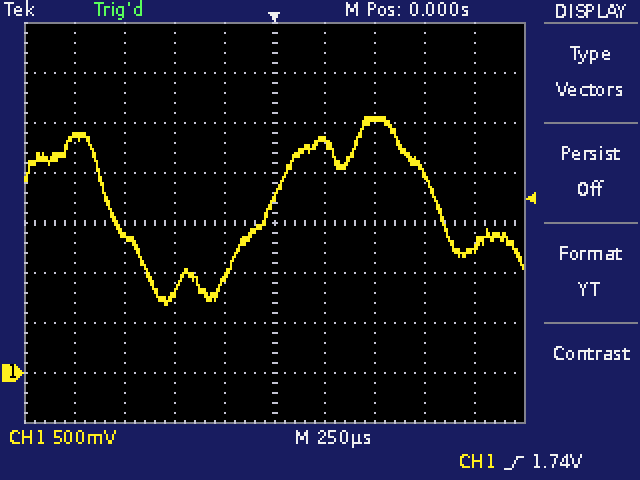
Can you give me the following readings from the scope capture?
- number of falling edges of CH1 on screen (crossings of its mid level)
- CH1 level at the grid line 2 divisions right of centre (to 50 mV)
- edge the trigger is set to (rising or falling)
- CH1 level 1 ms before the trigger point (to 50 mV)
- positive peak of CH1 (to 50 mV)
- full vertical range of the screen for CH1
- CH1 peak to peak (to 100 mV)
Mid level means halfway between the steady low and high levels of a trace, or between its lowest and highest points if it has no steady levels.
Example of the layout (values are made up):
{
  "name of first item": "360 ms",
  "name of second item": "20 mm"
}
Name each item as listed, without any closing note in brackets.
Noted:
{
  "number of falling edges of CH1 on screen": "2",
  "CH1 level at the grid line 2 divisions right of centre": "2.55 V",
  "edge the trigger is set to": "rising",
  "CH1 level 1 ms before the trigger point": "2.35 V",
  "positive peak of CH1": "2.55 V",
  "full vertical range of the screen for CH1": "4 V",
  "CH1 peak to peak": "1.90 V"
}
